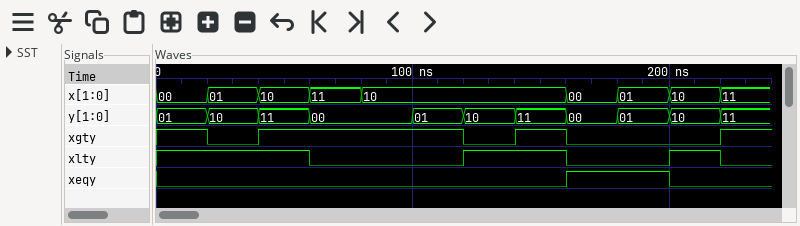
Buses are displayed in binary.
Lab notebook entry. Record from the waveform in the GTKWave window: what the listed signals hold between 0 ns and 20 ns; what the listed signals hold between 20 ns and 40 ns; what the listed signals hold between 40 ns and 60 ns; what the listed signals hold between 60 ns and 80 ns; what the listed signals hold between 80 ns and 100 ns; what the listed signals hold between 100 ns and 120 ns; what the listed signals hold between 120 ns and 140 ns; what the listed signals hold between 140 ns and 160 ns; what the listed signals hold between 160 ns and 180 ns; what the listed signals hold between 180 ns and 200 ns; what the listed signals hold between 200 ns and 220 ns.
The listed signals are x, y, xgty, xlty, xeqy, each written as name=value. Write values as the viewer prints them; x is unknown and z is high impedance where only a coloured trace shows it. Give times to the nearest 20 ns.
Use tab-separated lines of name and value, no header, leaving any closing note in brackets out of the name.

what the listed signals hold between 0 ns and 20 ns	x=00, y=01, xgty=1, xlty=1, xeqy=0
what the listed signals hold between 20 ns and 40 ns	x=01, y=10, xgty=0, xlty=1, xeqy=0
what the listed signals hold between 40 ns and 60 ns	x=10, y=11, xgty=1, xlty=1, xeqy=0
what the listed signals hold between 60 ns and 80 ns	x=11, y=00, xgty=1, xlty=0, xeqy=0
what the listed signals hold between 80 ns and 100 ns	x=10, y=00, xgty=1, xlty=0, xeqy=0
what the listed signals hold between 100 ns and 120 ns	x=10, y=01, xgty=1, xlty=0, xeqy=0
what the listed signals hold between 120 ns and 140 ns	x=10, y=10, xgty=0, xlty=1, xeqy=0
what the listed signals hold between 140 ns and 160 ns	x=10, y=11, xgty=1, xlty=1, xeqy=0
what the listed signals hold between 160 ns and 180 ns	x=00, y=00, xgty=0, xlty=0, xeqy=1
what the listed signals hold between 180 ns and 200 ns	x=01, y=01, xgty=0, xlty=0, xeqy=1
what the listed signals hold between 200 ns and 220 ns	x=10, y=10, xgty=0, xlty=1, xeqy=0
